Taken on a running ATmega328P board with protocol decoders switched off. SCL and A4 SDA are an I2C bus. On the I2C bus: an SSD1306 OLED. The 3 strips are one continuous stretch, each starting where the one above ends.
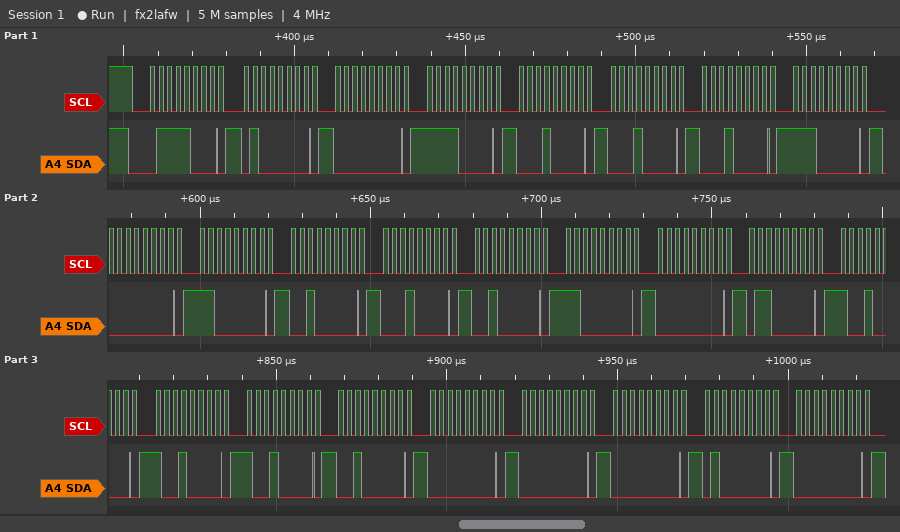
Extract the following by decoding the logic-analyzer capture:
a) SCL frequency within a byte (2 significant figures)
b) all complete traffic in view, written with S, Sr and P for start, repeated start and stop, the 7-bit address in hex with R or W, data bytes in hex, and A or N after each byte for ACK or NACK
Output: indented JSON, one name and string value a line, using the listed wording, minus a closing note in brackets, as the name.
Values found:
{
  "SCL frequency within a byte": "400 kHz",
  "all complete traffic in view, written with S, Sr and P for start, repeated start and stop, the 7-bit address in hex with R or W, data bytes in hex, and A or N after each byte for ACK or NACK": "S 3CW A 40 A 00 A F0 A 10 A 10 A 10 A E0 A 00 A C0 A 20 A 10 A 20 A C0 A 00 A 60 A 90 A 90 A 90 A 20 A 00 A 00 A 00 A 40 A 00 A"
}
